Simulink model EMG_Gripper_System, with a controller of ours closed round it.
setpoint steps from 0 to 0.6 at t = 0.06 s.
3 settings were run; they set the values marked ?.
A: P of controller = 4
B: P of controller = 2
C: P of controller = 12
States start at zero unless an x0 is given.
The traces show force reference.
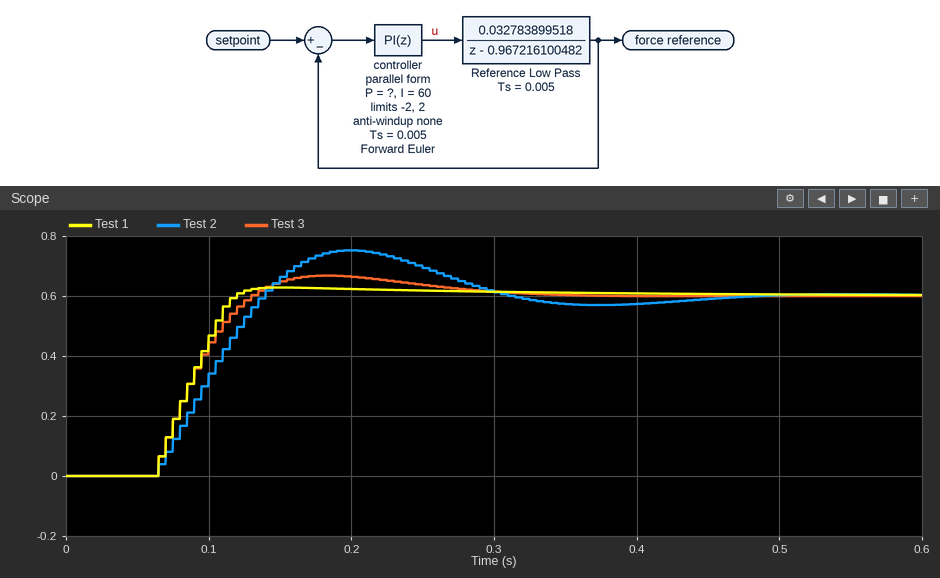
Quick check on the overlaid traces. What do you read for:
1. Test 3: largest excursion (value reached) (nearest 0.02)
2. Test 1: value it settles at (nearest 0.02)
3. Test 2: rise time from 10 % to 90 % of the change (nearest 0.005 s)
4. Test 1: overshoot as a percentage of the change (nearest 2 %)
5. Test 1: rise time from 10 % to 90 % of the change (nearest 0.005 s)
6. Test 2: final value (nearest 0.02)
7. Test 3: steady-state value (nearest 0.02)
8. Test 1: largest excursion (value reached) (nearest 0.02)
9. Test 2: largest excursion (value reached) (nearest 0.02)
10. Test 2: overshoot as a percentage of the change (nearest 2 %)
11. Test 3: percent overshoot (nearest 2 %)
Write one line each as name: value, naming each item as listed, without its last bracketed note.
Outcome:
Test 3: largest excursion (value reached): 0.66
Test 1: value it settles at: 0.60
Test 2: rise time from 10 % to 90 % of the change: 0.060 s
Test 1: overshoot as a percentage of the change: 4 %
Test 1: rise time from 10 % to 90 % of the change: 0.045 s
Test 2: final value: 0.60
Test 3: steady-state value: 0.60
Test 1: largest excursion (value reached): 0.62
Test 2: largest excursion (value reached): 0.76
Test 2: overshoot as a percentage of the change: 26 %
Test 3: percent overshoot: 12 %
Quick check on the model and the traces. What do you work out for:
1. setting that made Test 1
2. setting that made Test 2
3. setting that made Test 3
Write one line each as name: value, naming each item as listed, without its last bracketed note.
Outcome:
setting that made Test 1: C
setting that made Test 2: B
setting that made Test 3: A
